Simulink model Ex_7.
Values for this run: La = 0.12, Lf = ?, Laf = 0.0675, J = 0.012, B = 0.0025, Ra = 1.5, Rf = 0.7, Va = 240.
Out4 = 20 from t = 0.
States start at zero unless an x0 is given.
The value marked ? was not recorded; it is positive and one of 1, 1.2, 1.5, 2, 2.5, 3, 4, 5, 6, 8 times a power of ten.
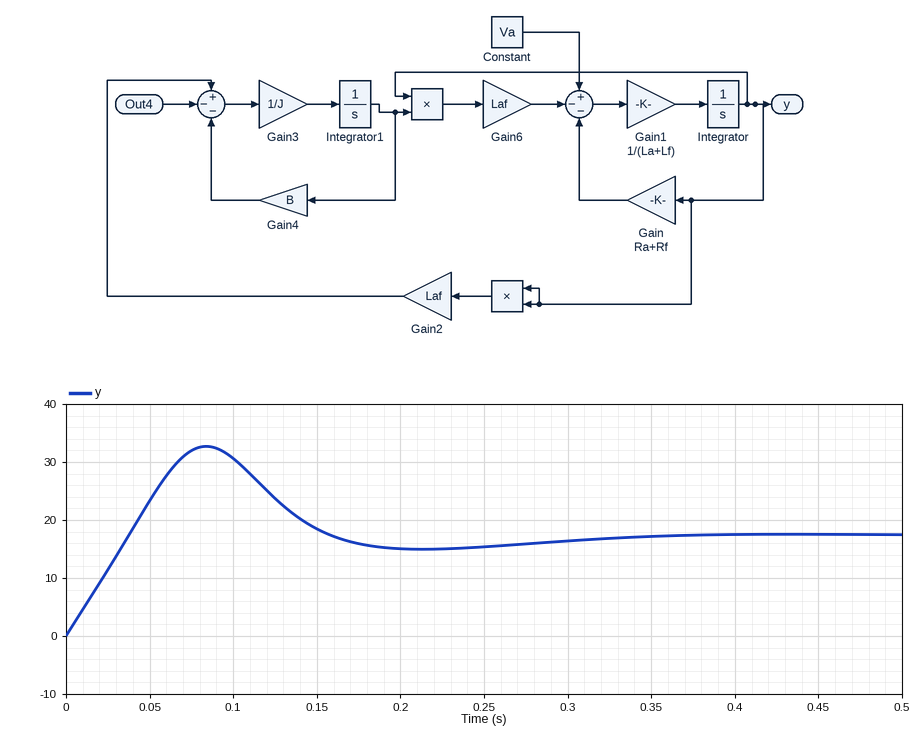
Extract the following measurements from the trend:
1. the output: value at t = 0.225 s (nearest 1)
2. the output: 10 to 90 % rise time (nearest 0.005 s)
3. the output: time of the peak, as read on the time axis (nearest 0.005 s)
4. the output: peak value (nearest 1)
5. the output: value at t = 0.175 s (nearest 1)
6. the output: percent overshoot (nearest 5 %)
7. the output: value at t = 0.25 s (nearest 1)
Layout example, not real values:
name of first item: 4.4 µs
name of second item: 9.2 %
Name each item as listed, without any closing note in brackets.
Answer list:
the output: value at t = 0.225 s: 15
the output: 10 to 90 % rise time: 0.030 s
the output: time of the peak, as read on the time axis: 0.085 s
the output: peak value: 33
the output: value at t = 0.175 s: 16
the output: percent overshoot: 90 %
the output: value at t = 0.25 s: 15
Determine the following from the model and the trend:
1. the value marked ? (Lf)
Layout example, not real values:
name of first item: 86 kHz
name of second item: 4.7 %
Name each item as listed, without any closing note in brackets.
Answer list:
the value marked ?: 0.4
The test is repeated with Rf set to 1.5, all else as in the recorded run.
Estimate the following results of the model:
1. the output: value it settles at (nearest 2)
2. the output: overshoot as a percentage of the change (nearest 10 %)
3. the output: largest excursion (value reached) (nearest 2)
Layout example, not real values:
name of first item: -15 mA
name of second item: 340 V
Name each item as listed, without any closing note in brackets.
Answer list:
the output: value it settles at: 18
the output: overshoot as a percentage of the change: 80 %
the output: largest excursion (value reached): 32
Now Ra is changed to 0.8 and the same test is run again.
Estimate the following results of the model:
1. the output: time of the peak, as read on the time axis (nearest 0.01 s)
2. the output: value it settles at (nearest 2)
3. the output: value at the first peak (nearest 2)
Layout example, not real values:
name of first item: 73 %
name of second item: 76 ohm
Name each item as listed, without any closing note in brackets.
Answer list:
the output: time of the peak, as read on the time axis: 0.08 s
the output: value it settles at: 18
the output: value at the first peak: 34
